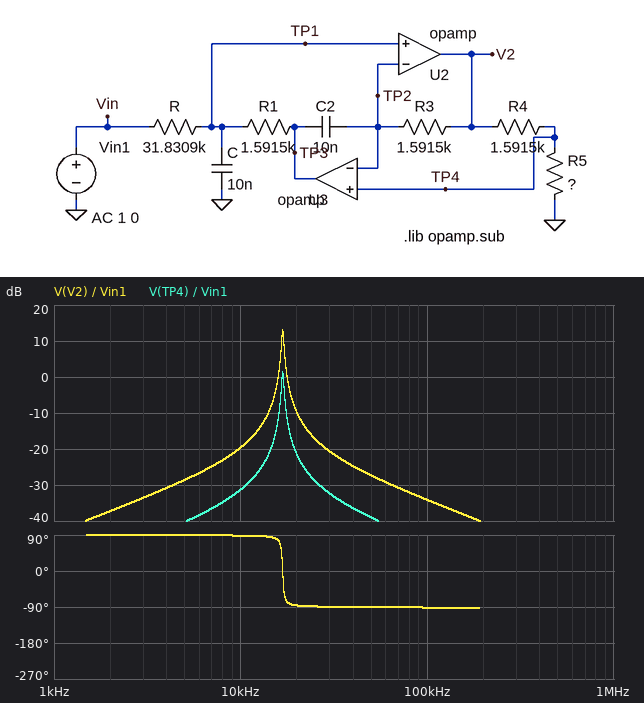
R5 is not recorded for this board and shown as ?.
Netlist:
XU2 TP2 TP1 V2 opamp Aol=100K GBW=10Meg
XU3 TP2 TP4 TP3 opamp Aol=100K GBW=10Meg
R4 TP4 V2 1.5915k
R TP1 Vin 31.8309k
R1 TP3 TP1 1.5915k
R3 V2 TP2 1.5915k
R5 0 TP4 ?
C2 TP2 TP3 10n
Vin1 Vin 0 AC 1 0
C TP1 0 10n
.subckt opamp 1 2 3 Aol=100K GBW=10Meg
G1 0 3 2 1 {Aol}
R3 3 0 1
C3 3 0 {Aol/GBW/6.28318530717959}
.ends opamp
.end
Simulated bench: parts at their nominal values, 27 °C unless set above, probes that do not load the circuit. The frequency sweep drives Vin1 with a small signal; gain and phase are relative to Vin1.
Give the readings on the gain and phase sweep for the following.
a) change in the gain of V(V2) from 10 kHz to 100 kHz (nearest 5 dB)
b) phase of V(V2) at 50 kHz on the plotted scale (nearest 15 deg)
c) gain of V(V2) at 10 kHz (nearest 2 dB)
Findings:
-15 dB
-90 deg
-20 dB
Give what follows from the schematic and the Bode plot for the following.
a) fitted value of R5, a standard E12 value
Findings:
560 Ω
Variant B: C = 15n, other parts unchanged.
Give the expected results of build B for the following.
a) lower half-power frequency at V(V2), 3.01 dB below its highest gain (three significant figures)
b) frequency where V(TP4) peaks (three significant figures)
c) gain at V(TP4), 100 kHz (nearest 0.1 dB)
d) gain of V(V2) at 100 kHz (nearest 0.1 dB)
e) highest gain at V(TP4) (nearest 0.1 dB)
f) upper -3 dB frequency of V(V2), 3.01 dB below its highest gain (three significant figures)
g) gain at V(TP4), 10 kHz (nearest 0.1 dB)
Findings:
13.6 kHz
13.7 kHz
-49.4 dB
-37.7 dB
1.3 dB
13.9 kHz
-28.5 dB
